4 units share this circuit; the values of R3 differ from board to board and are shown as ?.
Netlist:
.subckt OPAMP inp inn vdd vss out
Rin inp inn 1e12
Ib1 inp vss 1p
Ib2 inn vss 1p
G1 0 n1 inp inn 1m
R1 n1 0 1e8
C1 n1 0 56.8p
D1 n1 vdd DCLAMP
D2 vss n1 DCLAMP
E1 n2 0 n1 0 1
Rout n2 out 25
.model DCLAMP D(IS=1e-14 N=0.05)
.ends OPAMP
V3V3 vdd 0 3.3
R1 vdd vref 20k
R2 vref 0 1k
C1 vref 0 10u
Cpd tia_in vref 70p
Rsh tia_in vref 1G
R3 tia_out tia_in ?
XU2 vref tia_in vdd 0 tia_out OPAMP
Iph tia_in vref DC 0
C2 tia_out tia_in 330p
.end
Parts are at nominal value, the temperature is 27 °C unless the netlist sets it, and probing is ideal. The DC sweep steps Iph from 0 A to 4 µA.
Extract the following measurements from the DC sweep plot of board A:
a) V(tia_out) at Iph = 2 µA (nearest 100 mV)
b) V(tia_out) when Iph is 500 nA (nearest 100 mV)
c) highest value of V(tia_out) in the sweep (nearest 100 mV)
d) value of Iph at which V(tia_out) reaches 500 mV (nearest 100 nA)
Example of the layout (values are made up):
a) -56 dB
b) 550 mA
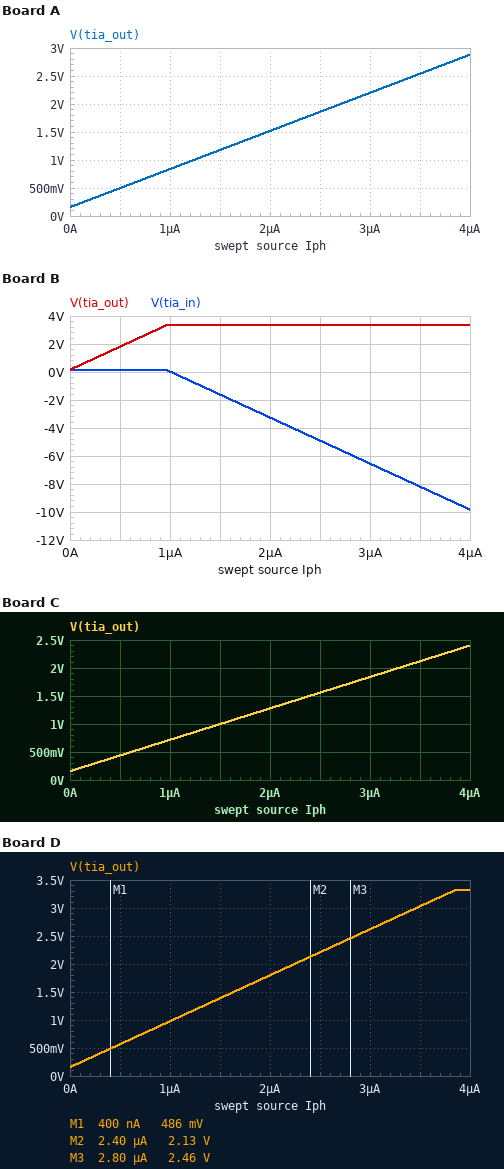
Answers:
a) 1.5 V
b) 500 mV
c) 2.9 V
d) 500 nA
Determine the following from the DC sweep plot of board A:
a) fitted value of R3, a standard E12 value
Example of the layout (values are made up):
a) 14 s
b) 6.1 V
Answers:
a) 680 kΩ
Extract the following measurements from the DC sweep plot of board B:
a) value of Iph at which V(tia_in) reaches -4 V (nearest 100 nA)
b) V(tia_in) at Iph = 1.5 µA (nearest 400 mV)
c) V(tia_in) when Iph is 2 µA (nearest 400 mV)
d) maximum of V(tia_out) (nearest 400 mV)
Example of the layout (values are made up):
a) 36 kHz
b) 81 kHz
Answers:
a) 2.2 µA
b) -1.6 V
c) -3.2 V
d) 3.2 V
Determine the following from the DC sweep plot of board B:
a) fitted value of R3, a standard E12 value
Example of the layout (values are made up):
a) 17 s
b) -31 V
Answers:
a) 3.3 MΩ
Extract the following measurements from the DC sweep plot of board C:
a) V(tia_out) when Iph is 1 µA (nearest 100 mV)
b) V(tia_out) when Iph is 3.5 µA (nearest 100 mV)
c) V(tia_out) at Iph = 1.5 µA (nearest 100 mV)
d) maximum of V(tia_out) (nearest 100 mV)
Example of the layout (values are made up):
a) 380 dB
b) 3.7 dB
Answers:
a) 700 mV
b) 2.1 V
c) 1.0 V
d) 2.4 V
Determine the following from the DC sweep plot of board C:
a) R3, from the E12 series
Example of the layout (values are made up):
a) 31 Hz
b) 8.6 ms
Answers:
a) 560 kΩ
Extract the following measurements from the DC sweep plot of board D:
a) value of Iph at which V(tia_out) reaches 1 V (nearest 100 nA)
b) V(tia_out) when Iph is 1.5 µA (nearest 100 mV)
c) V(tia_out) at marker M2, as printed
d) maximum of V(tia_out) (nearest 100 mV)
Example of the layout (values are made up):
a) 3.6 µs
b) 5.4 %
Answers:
a) 1.0 µA
b) 1.4 V
c) 2.13 V
d) 3.3 V
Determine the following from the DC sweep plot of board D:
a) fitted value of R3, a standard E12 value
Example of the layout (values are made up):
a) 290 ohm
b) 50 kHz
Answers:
a) 820 kΩ
